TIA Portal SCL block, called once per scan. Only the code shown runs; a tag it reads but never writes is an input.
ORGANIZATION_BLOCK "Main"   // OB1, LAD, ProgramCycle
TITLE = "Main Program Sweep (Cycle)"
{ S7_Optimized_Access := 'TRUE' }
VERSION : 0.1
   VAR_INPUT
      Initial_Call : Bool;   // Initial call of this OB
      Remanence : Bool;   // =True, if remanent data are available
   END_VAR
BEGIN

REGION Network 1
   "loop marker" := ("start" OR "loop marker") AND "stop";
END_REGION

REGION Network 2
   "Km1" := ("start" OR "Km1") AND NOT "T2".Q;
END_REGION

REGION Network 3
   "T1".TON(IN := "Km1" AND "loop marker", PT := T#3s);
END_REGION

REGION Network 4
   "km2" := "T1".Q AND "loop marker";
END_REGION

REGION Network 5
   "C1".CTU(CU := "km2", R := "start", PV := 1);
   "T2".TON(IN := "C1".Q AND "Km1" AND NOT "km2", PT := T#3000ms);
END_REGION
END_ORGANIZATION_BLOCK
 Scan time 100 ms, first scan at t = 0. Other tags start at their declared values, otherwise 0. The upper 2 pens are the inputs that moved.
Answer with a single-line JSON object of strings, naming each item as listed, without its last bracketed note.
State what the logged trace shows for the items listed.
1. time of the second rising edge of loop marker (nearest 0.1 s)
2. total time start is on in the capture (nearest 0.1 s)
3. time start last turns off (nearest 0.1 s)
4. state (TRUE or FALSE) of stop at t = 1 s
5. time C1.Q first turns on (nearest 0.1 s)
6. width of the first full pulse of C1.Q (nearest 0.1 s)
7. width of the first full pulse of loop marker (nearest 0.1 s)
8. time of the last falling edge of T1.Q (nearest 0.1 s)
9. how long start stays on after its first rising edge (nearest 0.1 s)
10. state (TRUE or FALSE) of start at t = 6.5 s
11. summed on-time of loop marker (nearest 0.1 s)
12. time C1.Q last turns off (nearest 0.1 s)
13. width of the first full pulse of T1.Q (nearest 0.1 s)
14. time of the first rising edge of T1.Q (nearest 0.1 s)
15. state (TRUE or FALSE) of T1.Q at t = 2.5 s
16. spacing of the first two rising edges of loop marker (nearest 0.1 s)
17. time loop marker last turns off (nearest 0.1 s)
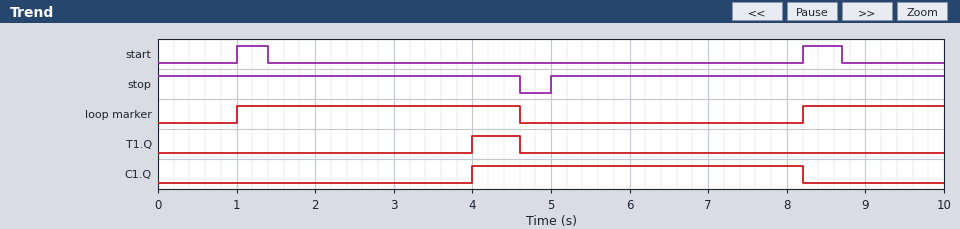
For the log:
{"time of the second rising edge of loop marker": "8.2 s", "total time start is on in the capture": "0.9 s", "time start last turns off": "8.7 s", "state (TRUE or FALSE) of stop at t = 1 s": "TRUE", "time C1.Q first turns on": "4.0 s", "width of the first full pulse of C1.Q": "4.2 s", "width of the first full pulse of loop marker": "3.6 s", "time of the last falling edge of T1.Q": "4.6 s", "how long start stays on after its first rising edge": "0.4 s", "state (TRUE or FALSE) of start at t = 6.5 s": "FALSE", "summed on-time of loop marker": "5.4 s", "time C1.Q last turns off": "8.2 s", "width of the first full pulse of T1.Q": "0.6 s", "time of the first rising edge of T1.Q": "4.0 s", "state (TRUE or FALSE) of T1.Q at t = 2.5 s": "FALSE", "spacing of the first two rising edges of loop marker": "7.2 s", "time loop marker last turns off": "4.6 s"}
